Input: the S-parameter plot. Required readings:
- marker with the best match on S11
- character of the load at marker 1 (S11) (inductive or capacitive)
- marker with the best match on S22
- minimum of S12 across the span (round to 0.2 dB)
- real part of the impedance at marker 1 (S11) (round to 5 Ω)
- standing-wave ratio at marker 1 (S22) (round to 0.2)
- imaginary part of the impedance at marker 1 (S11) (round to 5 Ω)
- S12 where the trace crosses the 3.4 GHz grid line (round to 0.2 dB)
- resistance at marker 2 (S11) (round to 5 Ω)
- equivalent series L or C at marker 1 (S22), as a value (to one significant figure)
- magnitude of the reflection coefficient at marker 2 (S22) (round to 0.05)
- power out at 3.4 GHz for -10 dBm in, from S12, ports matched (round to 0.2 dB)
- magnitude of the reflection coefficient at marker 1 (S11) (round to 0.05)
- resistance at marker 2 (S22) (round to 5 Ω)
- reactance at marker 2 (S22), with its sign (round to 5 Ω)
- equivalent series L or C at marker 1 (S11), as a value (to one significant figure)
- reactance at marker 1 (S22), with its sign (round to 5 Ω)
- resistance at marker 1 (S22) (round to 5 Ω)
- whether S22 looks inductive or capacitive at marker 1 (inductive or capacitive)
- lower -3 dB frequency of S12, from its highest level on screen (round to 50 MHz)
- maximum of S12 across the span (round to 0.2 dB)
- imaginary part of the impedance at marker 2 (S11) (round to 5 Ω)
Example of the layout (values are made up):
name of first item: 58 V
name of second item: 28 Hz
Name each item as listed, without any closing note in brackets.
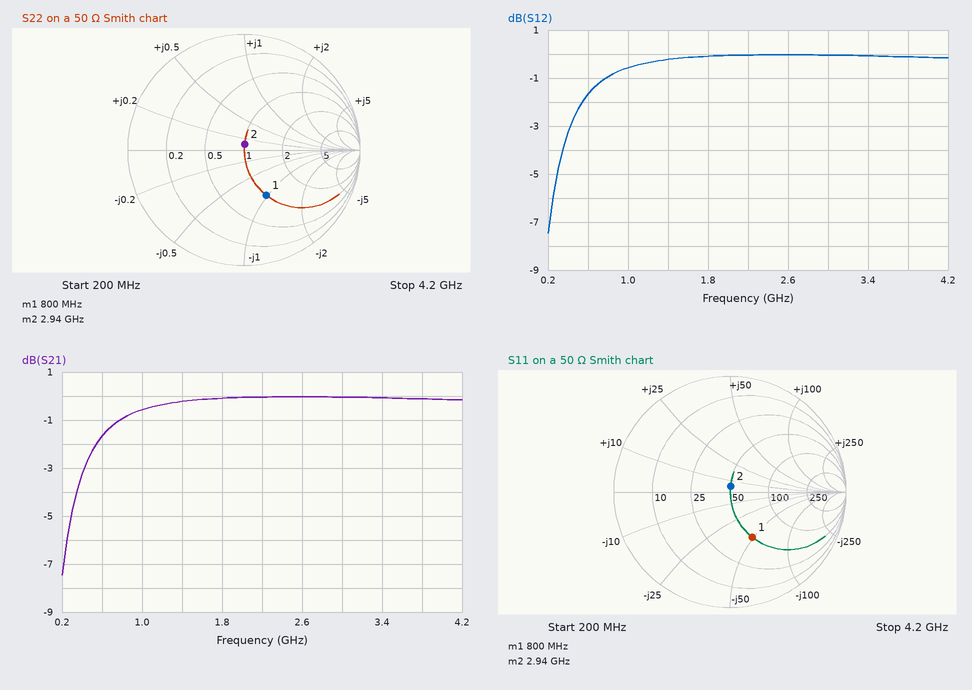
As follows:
marker with the best match on S11: marker 2
character of the load at marker 1 (S11): capacitive
marker with the best match on S22: marker 2
minimum of S12 across the span: -7.4 dB
real part of the impedance at marker 1 (S11): 50 Ω
standing-wave ratio at marker 1 (S22): 2.6
imaginary part of the impedance at marker 1 (S11): -50 Ω
S12 where the trace crosses the 3.4 GHz grid line: 0.0 dB
resistance at marker 2 (S11): 50 Ω
equivalent series L or C at marker 1 (S22), as a value: 4 pF
magnitude of the reflection coefficient at marker 2 (S22): 0.05
power out at 3.4 GHz for -10 dBm in, from S12, ports matched: -10.0 dBm
magnitude of the reflection coefficient at marker 1 (S11): 0.45
resistance at marker 2 (S22): 50 Ω
reactance at marker 2 (S22), with its sign: +5 Ω
equivalent series L or C at marker 1 (S11), as a value: 4 pF
reactance at marker 1 (S22), with its sign: -50 Ω
resistance at marker 1 (S22): 50 Ω
whether S22 looks inductive or capacitive at marker 1: capacitive
lower -3 dB frequency of S12, from its highest level on screen: 400 MHz
maximum of S12 across the span: 0.0 dB
imaginary part of the impedance at marker 2 (S11): +5 Ω
